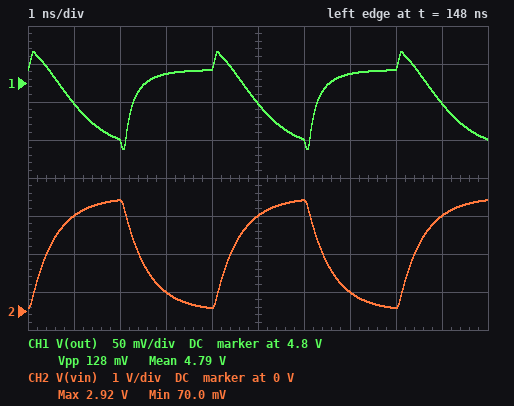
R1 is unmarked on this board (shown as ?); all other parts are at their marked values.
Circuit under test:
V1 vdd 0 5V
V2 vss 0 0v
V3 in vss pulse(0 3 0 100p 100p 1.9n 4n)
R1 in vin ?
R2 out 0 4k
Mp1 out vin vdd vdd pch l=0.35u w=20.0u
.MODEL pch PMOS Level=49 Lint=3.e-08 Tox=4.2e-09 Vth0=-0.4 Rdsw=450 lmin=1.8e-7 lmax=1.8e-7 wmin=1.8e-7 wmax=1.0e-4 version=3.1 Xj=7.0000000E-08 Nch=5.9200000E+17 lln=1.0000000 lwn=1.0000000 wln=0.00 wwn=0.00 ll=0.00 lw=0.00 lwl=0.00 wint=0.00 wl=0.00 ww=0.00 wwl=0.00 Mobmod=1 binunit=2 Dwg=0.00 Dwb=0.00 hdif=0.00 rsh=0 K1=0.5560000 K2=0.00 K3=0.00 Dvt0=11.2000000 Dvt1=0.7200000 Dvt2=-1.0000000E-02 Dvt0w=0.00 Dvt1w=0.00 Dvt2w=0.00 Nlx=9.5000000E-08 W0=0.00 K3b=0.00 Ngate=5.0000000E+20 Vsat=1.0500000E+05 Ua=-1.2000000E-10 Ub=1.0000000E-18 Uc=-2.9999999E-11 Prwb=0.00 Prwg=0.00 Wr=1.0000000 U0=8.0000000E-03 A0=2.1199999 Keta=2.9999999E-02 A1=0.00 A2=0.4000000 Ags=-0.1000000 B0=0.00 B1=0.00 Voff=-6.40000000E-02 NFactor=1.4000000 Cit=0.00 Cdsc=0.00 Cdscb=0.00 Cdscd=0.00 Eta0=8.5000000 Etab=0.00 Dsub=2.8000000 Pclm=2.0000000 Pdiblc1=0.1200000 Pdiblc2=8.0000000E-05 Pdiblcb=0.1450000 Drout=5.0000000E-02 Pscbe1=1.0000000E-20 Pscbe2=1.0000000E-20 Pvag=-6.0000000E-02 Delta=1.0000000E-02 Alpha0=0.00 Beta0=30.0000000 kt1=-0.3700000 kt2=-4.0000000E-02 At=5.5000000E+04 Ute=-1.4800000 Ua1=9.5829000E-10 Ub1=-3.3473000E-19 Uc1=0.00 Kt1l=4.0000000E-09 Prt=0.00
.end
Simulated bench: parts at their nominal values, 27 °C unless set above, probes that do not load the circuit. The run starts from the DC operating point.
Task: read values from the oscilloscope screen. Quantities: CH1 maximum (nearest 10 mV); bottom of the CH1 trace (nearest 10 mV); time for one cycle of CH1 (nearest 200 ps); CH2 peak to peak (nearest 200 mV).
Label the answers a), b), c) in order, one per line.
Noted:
a) 4.84 V
b) 4.71 V
c) 4.0 ns
d) 2.8 V
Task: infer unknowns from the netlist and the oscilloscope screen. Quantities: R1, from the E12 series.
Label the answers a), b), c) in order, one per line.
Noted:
a) 8.2 kΩ
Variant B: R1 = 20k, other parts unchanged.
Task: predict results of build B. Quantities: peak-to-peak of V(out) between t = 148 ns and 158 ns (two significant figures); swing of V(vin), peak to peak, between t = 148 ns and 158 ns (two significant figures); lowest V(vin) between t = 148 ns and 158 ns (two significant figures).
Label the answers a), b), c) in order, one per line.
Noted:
a) 62 mV
b) 1.9 V
c) 540 mV
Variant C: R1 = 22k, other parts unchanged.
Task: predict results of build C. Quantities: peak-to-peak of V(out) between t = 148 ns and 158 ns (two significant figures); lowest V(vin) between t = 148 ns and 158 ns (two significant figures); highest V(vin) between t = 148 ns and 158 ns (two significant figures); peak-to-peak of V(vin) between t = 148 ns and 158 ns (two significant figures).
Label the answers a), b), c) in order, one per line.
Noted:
a) 56 mV
b) 610 mV
c) 2.4 V
d) 1.8 V
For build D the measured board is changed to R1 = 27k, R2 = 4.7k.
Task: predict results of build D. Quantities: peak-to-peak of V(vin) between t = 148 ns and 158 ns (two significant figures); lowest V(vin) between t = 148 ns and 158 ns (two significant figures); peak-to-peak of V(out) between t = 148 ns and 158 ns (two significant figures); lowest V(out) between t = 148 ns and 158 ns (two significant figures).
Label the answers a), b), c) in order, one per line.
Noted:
a) 1.5 V
b) 740 mV
c) 39 mV
d) 4.8 V
